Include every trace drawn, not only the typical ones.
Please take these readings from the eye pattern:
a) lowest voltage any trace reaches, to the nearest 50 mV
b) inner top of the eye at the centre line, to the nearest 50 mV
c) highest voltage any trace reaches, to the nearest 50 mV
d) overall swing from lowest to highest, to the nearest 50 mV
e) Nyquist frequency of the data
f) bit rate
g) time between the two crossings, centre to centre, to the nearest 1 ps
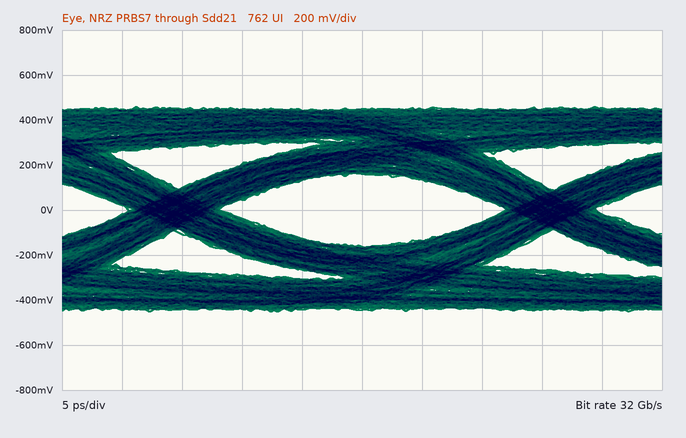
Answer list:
-450 mV
150 mV
450 mV
900 mV
16 GHz
32 Gb/s
31 ps
